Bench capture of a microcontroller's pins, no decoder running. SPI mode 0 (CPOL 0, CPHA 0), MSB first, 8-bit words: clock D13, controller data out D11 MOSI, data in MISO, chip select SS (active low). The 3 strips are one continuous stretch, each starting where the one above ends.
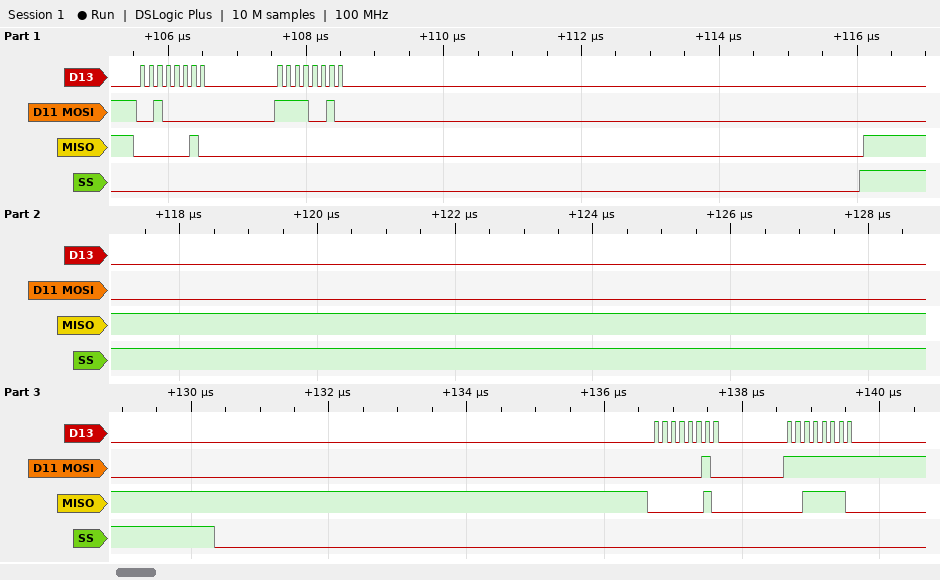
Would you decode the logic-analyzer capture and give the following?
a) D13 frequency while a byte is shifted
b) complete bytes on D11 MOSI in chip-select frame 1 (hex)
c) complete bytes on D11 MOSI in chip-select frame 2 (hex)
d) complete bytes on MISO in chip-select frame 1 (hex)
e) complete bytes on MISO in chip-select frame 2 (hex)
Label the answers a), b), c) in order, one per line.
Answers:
a) 8 MHz
b) 20 F2
c) 02 FF
d) 02 00
e) 02 3E
